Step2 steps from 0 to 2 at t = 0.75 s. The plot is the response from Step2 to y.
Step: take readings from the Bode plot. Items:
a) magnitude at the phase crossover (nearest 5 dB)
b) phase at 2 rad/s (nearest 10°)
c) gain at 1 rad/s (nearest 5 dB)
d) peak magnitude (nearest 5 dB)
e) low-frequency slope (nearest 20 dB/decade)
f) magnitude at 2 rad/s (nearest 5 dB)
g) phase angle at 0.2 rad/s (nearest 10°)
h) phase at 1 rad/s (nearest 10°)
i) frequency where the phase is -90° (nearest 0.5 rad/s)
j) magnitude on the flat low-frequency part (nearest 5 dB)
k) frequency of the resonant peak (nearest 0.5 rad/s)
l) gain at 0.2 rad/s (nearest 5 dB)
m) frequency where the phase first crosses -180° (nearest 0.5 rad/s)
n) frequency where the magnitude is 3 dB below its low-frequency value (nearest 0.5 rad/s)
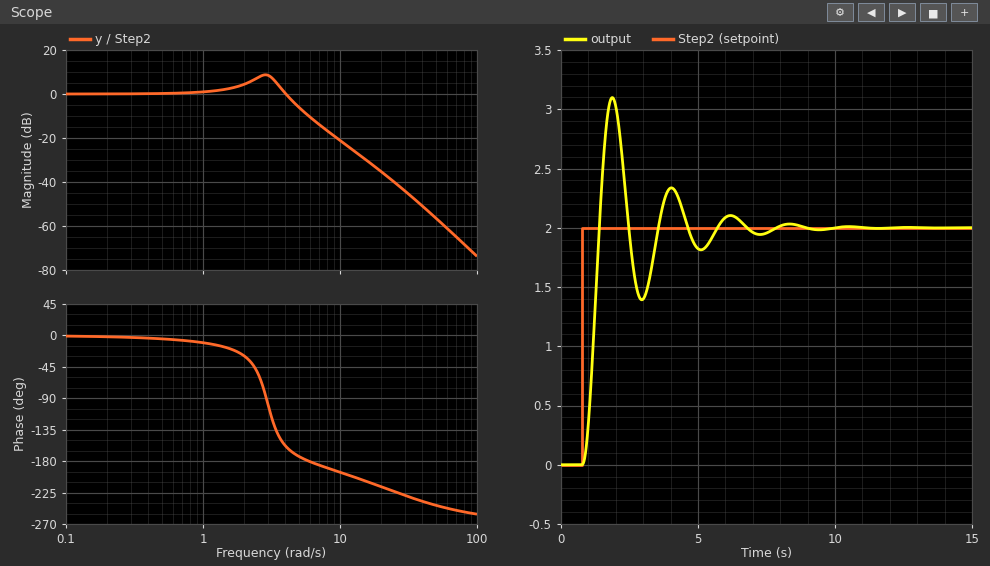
-10 dB
-30°
0 dB
10 dB
0 dB/decade
5 dB
0°
-10°
3.0 rad/s
0 dB
3.0 rad/s
0 dB
6.0 rad/s
4.5 rad/s
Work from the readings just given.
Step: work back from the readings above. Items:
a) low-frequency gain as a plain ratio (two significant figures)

1.0
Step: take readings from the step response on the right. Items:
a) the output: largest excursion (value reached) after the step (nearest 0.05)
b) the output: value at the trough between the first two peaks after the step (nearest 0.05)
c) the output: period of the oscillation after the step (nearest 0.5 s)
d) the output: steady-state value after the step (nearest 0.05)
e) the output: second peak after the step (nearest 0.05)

3.10
1.40
2.0 s
2.00
2.35
